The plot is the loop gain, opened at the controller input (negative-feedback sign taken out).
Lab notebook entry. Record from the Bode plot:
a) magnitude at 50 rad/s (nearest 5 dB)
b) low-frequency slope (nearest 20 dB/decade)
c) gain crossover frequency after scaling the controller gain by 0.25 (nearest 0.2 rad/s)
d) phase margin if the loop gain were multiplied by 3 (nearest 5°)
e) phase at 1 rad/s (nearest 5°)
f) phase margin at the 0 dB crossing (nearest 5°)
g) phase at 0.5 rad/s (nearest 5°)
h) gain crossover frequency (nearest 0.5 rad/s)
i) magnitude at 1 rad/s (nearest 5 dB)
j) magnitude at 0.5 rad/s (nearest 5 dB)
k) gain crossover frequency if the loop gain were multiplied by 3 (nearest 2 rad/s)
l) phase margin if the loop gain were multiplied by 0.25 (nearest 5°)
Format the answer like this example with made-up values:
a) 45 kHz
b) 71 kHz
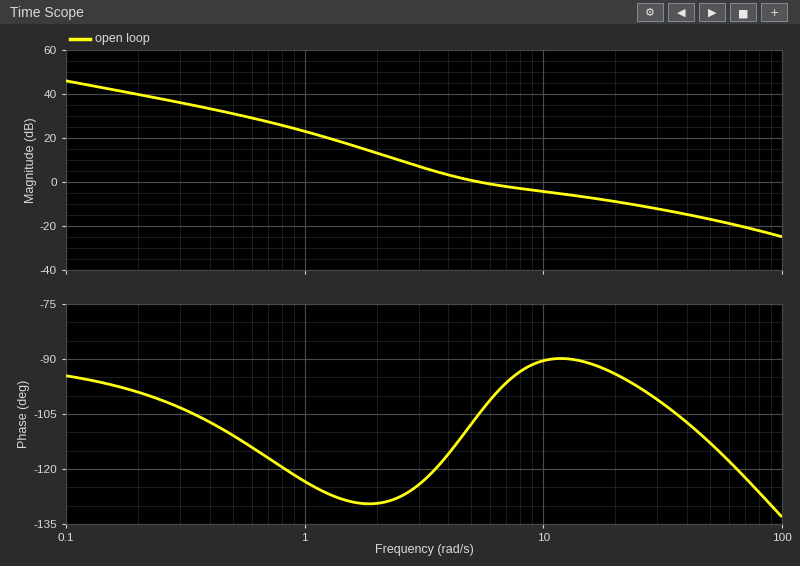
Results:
a) -15 dB
b) -20 dB/decade
c) 2.2 rad/s
d) 85°
e) -125°
f) 75°
g) -110°
h) 5.5 rad/s
i) 25 dB
j) 30 dB
k) 22 rad/s
l) 50°
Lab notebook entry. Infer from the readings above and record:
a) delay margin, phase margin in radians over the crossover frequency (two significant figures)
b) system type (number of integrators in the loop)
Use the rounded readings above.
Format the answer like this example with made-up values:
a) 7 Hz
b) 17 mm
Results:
a) 0.24 s
b) 1
